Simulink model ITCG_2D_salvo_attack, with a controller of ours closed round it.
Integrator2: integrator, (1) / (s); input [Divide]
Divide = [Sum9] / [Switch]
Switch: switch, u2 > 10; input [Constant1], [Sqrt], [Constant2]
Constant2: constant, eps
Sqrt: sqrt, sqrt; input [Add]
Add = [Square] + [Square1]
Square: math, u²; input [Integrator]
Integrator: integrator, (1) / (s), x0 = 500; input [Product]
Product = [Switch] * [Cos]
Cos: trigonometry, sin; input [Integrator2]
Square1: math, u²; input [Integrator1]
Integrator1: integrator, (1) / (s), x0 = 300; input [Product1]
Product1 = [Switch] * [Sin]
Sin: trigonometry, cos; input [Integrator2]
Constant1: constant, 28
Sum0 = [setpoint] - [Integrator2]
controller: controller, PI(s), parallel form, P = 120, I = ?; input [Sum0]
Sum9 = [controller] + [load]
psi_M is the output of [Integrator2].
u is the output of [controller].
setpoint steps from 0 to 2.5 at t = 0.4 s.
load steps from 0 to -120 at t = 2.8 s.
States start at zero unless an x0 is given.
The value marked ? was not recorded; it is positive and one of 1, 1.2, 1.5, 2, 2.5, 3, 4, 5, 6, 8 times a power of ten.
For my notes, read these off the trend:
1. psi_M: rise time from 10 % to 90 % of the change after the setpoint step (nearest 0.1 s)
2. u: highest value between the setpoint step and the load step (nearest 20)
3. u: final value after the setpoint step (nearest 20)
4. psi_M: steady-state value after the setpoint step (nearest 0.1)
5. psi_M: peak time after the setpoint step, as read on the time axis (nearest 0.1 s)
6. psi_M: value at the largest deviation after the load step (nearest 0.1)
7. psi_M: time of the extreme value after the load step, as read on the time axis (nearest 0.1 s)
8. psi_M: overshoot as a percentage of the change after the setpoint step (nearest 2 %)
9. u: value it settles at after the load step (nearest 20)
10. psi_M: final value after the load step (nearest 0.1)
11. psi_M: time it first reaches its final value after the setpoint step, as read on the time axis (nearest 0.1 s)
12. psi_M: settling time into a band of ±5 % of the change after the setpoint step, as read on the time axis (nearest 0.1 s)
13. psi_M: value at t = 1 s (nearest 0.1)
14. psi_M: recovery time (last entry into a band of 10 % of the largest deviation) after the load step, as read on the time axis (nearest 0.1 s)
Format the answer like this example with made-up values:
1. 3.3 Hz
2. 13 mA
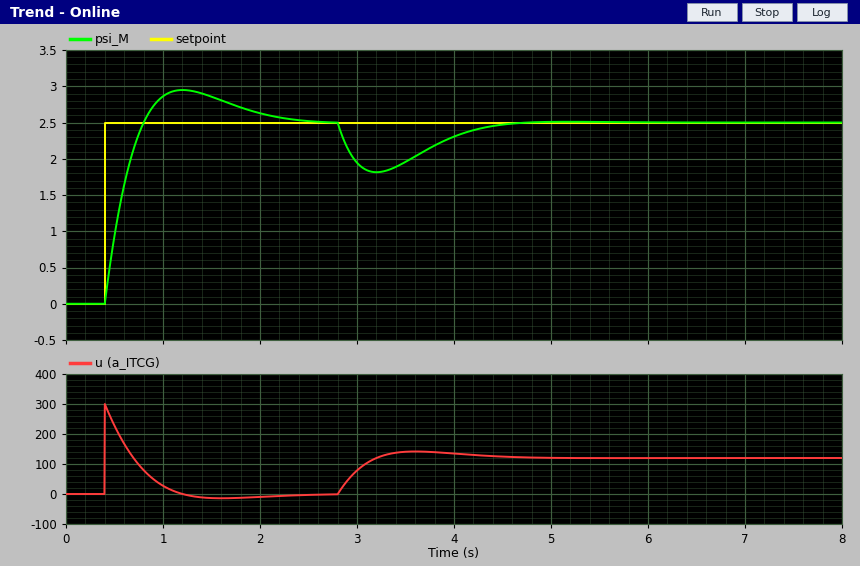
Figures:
1. 0.3 s
2. 300
3. 0
4. 2.5
5. 1.2 s
6. 1.8
7. 3.2 s
8. 18 %
9. 120
10. 2.5
11. 0.8 s
12. 2.0 s
13. 2.9
14. 4.3 s
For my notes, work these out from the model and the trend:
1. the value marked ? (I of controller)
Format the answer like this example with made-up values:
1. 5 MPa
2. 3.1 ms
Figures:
1. 200
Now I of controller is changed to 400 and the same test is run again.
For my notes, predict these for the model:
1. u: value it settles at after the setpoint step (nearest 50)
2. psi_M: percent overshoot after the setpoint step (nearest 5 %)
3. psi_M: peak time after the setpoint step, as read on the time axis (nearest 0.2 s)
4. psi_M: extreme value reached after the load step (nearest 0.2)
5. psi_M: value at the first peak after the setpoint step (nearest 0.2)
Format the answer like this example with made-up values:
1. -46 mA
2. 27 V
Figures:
1. 0
2. 25 %
3. 1.0 s
4. 2.0
5. 3.2
